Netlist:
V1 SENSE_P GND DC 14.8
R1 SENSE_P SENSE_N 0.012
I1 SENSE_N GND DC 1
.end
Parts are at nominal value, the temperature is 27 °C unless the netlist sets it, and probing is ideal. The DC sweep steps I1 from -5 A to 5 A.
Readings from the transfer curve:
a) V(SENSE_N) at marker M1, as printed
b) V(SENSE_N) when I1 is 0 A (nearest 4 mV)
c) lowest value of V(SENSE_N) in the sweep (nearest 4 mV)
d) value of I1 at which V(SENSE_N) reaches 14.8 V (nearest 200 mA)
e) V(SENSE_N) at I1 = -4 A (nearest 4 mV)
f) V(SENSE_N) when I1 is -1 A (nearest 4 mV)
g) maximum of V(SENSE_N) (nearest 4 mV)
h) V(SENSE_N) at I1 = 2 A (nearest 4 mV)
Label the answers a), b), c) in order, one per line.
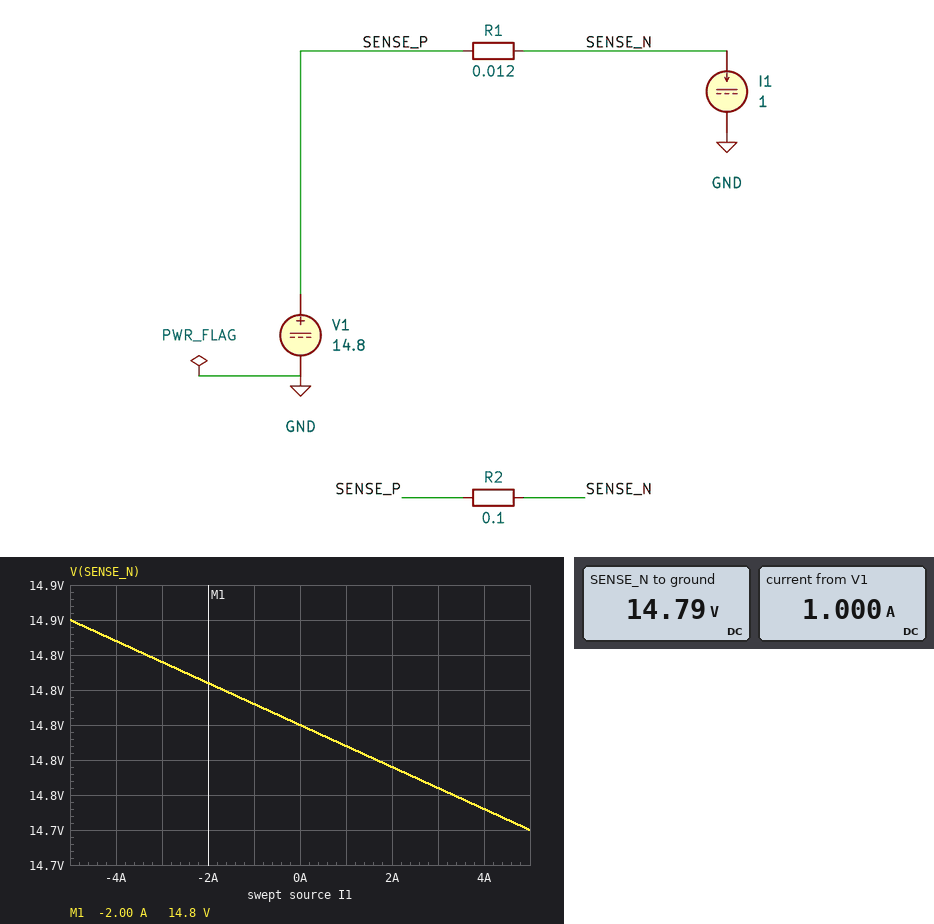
a) 14.8 V
b) 14.800 V
c) 14.740 V
d) 0 A
e) 14.848 V
f) 14.812 V
g) 14.860 V
h) 14.776 V
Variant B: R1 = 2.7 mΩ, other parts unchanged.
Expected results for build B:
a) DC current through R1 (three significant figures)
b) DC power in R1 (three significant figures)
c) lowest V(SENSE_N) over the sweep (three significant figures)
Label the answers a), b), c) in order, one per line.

a) 1.00 A
b) 2.70 mW
c) 14.8 V
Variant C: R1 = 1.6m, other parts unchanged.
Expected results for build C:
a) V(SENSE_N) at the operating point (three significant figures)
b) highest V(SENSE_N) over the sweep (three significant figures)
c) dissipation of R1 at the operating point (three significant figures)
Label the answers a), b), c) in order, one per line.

a) 14.8 V
b) 14.8 V
c) 1.60 mW
